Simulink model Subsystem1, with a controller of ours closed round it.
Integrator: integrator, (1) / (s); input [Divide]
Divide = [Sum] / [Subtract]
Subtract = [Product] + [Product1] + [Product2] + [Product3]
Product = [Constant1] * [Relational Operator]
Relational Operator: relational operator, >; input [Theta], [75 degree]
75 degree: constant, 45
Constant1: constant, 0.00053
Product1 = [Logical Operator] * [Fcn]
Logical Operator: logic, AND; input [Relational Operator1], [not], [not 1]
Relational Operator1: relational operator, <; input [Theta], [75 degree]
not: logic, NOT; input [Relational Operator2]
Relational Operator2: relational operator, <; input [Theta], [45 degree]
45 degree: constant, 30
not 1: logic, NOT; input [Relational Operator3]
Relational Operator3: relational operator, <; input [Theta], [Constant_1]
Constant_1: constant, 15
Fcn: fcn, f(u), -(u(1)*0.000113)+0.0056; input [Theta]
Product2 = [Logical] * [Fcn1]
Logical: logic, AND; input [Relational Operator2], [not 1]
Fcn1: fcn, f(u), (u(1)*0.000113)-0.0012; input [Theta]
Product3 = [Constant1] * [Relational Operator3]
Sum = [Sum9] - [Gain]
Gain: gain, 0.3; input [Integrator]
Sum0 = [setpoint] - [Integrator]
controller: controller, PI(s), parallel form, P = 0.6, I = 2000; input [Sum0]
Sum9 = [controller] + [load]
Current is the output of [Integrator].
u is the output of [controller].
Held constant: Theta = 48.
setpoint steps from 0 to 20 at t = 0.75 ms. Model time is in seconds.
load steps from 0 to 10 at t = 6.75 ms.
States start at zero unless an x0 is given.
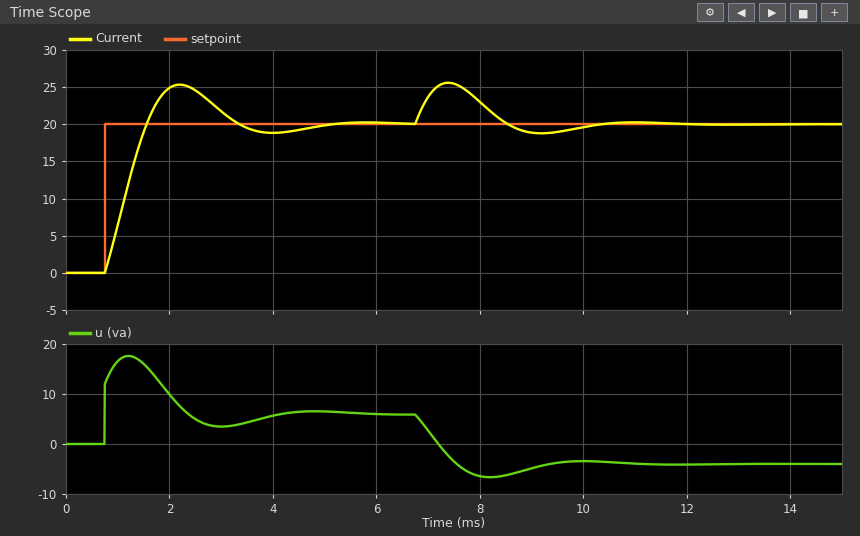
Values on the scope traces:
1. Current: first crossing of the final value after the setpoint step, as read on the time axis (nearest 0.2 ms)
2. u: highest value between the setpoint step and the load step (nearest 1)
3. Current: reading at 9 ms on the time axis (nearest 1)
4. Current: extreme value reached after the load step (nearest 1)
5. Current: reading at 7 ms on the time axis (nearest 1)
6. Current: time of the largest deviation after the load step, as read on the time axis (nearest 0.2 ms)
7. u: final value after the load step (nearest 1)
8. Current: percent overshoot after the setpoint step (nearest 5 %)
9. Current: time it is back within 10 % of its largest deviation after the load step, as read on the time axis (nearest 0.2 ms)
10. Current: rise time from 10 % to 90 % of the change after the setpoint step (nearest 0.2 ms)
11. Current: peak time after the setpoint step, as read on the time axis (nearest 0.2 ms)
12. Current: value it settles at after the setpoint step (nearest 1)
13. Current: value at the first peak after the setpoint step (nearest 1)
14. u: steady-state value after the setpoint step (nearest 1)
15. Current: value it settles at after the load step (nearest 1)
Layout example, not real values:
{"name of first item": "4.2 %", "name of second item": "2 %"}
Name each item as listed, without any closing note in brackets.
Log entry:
{"Current: first crossing of the final value after the setpoint step, as read on the time axis": "1.6 ms", "u: highest value between the setpoint step and the load step": "18", "Current: reading at 9 ms on the time axis": "19", "Current: extreme value reached after the load step": "26", "Current: reading at 7 ms on the time axis": "24", "Current: time of the largest deviation after the load step, as read on the time axis": "7.4 ms", "u: final value after the load step": "-4", "Current: percent overshoot after the setpoint step": "25 %", "Current: time it is back within 10 % of its largest deviation after the load step, as read on the time axis": "9.8 ms", "Current: rise time from 10 % to 90 % of the change after the setpoint step": "0.6 ms", "Current: peak time after the setpoint step, as read on the time axis": "2.2 ms", "Current: value it settles at after the setpoint step": "20", "Current: value at the first peak after the setpoint step": "25", "u: steady-state value after the setpoint step": "6", "Current: value it settles at after the load step": "20"}
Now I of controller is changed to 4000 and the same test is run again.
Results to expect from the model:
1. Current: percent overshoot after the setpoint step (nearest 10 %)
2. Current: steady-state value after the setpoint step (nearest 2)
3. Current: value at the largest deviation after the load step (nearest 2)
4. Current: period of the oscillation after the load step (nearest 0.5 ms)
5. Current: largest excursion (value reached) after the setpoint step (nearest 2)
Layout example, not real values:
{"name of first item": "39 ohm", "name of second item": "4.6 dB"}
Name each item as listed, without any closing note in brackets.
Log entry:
{"Current: percent overshoot after the setpoint step": "40 %", "Current: steady-state value after the setpoint step": "20", "Current: value at the largest deviation after the load step": "24", "Current: period of the oscillation after the load step": "2.5 ms", "Current: largest excursion (value reached) after the setpoint step": "28"}
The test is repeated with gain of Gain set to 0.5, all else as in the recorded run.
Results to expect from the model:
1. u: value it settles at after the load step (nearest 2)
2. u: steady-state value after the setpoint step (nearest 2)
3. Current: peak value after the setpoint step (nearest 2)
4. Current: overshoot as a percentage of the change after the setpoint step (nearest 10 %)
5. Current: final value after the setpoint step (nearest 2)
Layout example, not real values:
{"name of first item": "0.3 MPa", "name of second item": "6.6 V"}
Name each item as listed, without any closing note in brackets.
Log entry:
{"u: value it settles at after the load step": "0", "u: steady-state value after the setpoint step": "10", "Current: peak value after the setpoint step": "24", "Current: overshoot as a percentage of the change after the setpoint step": "20 %", "Current: final value after the setpoint step": "20"}
